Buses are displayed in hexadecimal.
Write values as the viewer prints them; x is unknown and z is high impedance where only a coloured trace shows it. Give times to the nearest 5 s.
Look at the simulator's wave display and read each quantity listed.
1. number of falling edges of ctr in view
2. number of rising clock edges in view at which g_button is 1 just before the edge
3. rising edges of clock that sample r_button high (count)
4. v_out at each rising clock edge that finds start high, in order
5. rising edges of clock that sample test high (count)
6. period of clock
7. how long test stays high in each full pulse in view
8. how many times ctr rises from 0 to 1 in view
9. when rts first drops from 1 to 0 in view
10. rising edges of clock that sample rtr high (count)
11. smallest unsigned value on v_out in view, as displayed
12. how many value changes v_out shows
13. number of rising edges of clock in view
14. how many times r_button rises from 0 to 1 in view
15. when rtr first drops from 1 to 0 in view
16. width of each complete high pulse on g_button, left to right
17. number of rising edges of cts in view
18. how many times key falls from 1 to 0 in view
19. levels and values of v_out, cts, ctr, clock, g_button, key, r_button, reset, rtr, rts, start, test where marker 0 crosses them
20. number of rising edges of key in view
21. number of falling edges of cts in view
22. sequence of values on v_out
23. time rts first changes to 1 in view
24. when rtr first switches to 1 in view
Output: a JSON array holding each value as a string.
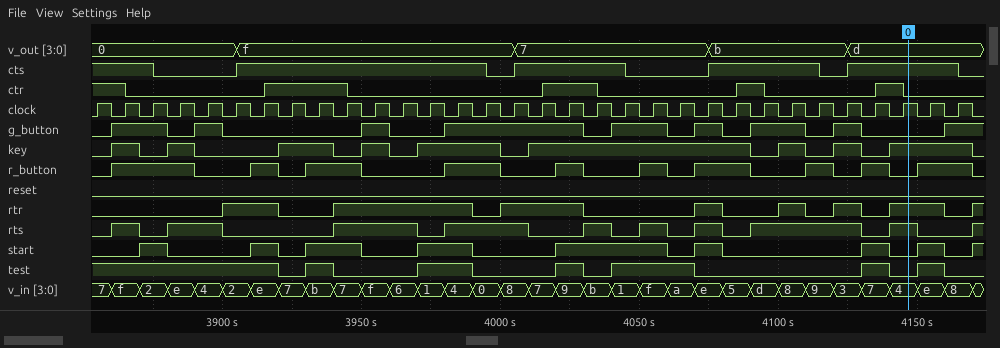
["5", "16", "16", "0, f, f, f, f, f, 7, 7, 7, 7, 7, d, d", "16", "10 s", "10 s, 20 s, 10 s, 30 s, 10 s, 10 s", "4", "3870 s", "15", "0", "4", "32", "10", "3920 s", "20 s, 10 s, 10 s, 50 s, 20 s, 10 s, 20 s, 10 s", "4", "9", "v_out=d, cts=1, ctr=0, clock=1, g_button=0, key=1, r_button=0, reset=0, rtr=1, rts=1, start=0, test=0", "9", "5", "0, f, 7, b, d", "3860 s", "3900 s"]
